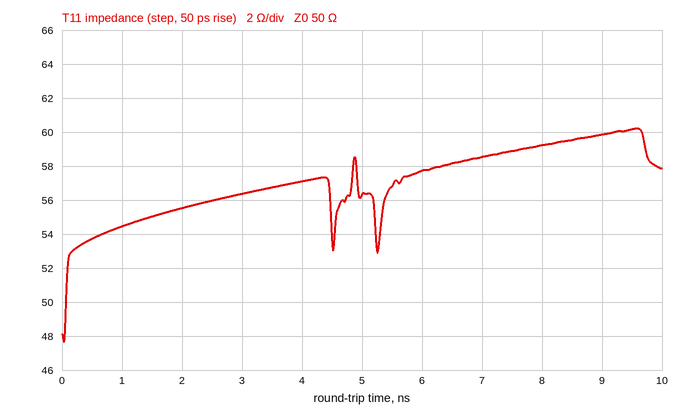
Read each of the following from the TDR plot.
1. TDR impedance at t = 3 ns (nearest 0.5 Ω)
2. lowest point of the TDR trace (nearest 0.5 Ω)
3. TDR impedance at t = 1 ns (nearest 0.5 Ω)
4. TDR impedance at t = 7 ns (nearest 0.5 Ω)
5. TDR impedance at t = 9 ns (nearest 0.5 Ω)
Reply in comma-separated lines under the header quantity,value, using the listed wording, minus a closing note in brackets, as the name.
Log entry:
quantity,value
TDR impedance at t = 3 ns,56.5 Ω
lowest point of the TDR trace,47.5 Ω
TDR impedance at t = 1 ns,54.5 Ω
TDR impedance at t = 7 ns,58.5 Ω
TDR impedance at t = 9 ns,60.0 Ω
